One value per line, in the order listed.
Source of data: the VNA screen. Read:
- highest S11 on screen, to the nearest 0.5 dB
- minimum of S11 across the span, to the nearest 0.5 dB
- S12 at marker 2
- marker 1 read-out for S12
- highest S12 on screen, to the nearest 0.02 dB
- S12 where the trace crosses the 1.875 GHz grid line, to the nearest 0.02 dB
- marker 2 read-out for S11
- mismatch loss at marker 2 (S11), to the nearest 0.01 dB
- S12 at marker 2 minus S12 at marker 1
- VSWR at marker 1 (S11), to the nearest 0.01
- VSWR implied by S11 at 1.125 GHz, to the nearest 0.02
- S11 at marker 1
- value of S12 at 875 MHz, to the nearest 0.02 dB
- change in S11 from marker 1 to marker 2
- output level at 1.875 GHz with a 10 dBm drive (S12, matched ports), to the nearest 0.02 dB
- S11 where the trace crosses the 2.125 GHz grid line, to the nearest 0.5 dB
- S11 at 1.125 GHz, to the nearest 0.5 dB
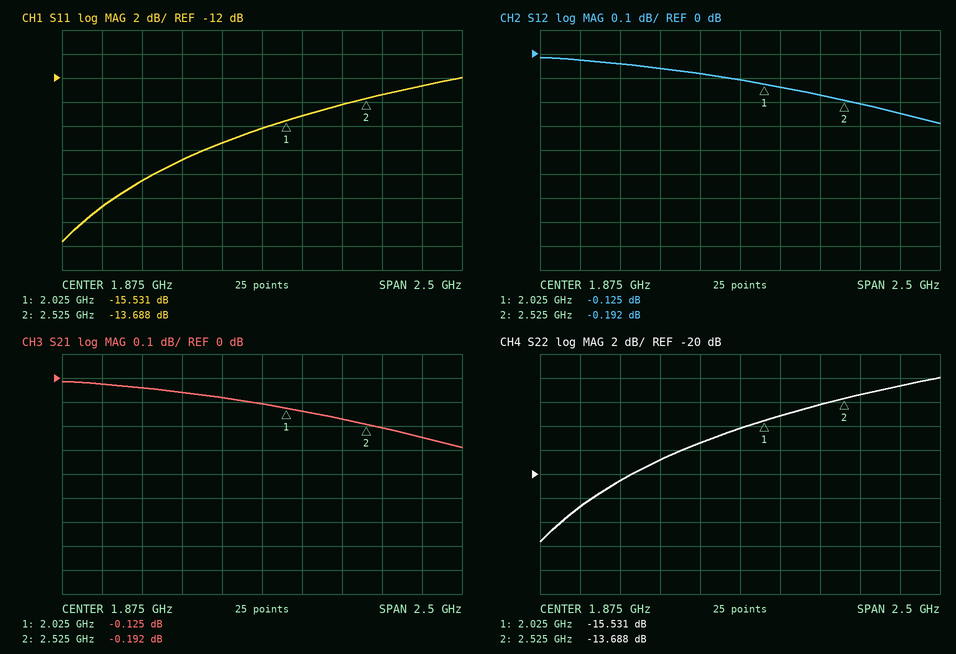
-12.0 dB
-25.5 dB
-0.192 dB
-0.125 dB
-0.02 dB
-0.10 dB
-13.688 dB
0.19 dB
-0.067 dB
1.40
1.20
-15.531 dB
-0.02 dB
1.843 dB
9.90 dBm
-15.0 dB
-20.5 dB
